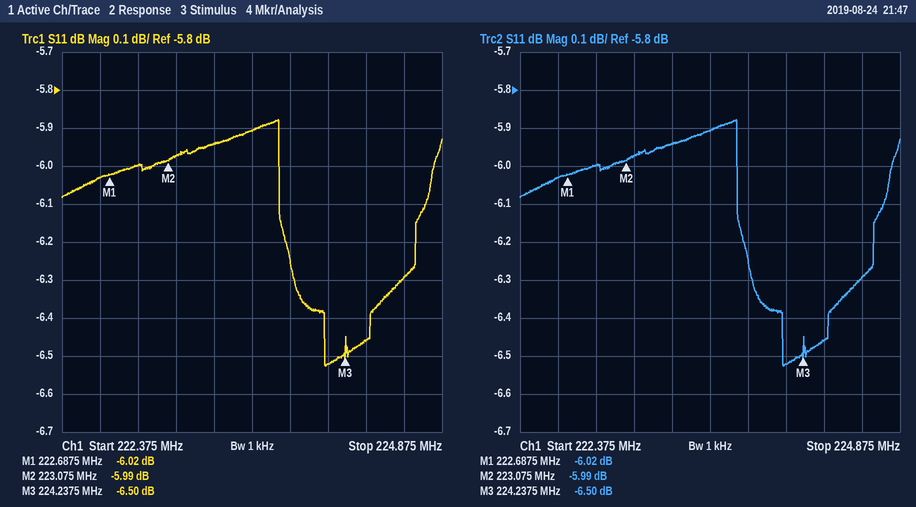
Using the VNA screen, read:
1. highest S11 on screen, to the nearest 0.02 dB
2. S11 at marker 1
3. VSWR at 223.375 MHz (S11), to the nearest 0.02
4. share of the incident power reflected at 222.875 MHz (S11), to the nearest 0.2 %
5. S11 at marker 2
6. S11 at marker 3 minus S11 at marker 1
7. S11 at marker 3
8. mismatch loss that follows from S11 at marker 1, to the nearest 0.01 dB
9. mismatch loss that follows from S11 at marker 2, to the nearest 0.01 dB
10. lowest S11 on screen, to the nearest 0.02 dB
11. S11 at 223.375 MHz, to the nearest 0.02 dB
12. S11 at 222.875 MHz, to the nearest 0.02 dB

-5.88 dB
-6.02 dB
3.04
25.2 %
-5.99 dB
-0.48 dB
-6.50 dB
1.25 dB
1.26 dB
-6.52 dB
-5.94 dB
-6.00 dB
